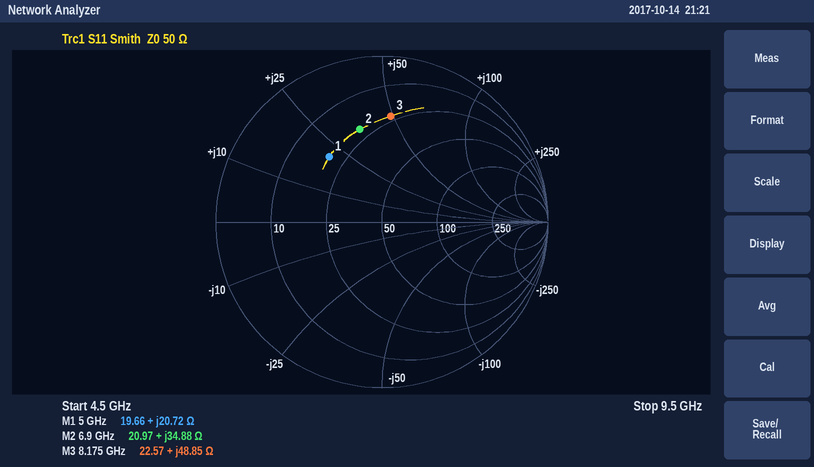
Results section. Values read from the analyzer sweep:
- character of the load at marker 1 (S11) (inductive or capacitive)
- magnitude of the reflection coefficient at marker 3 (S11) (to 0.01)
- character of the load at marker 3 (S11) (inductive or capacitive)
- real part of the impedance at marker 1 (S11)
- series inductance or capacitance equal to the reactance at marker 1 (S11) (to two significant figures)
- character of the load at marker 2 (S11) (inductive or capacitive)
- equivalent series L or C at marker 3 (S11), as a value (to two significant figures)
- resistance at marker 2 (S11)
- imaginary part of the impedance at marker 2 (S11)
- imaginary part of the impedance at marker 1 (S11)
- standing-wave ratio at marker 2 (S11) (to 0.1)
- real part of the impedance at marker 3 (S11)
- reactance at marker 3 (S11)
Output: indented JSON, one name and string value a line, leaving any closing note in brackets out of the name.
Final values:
{
  "character of the load at marker 1 (S11)": "inductive",
  "magnitude of the reflection coefficient at marker 3 (S11)": "0.64",
  "character of the load at marker 3 (S11)": "inductive",
  "real part of the impedance at marker 1": "19.66 Ω",
  "series inductance or capacitance equal to the reactance at marker 1 (S11)": "660 pH",
  "character of the load at marker 2 (S11)": "inductive",
  "equivalent series L or C at marker 3 (S11), as a value": "950 pH",
  "resistance at marker 2": "20.97 Ω",
  "imaginary part of the impedance at marker 2": "+34.88 Ω",
  "imaginary part of the impedance at marker 1": "+20.72 Ω",
  "standing-wave ratio at marker 2 (S11)": "3.7",
  "real part of the impedance at marker 3": "22.57 Ω",
  "reactance at marker 3": "+48.85 Ω"
}
